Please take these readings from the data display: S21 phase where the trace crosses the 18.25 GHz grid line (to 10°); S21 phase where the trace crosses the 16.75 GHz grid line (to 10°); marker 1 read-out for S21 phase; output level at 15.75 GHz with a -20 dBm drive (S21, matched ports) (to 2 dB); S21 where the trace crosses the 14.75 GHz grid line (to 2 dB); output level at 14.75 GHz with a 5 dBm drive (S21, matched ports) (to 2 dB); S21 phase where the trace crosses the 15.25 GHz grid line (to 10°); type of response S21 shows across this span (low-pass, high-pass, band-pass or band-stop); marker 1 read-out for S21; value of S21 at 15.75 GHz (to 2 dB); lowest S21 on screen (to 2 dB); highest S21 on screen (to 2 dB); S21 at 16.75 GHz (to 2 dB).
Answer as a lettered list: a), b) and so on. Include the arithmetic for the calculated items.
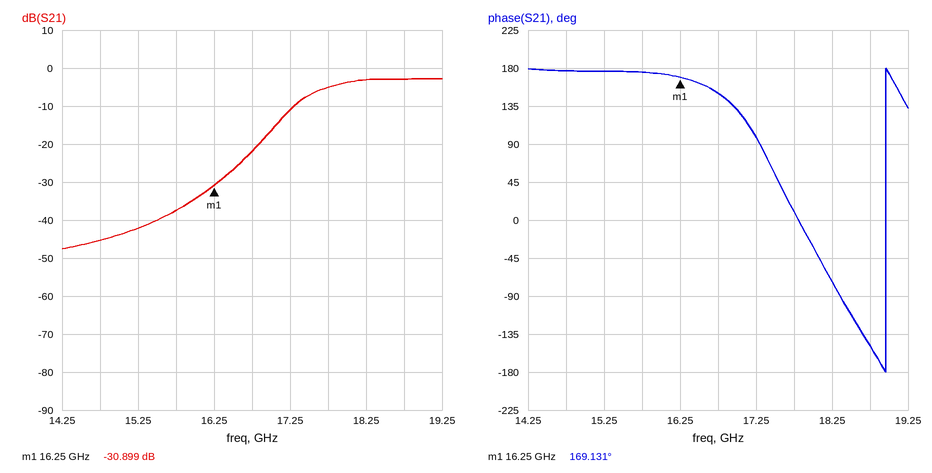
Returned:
a) -70°
b) 150°
c) 169.131°
d) -20 dBm + (-38 dB) = -58 dBm
e) -46 dB
f) 5 dBm + (-46 dB) = -40 dBm
g) 180°
h) high-pass
i) -30.899 dB
j) -38 dB
k) -48 dB
l) -2 dB
m) -22 dB
